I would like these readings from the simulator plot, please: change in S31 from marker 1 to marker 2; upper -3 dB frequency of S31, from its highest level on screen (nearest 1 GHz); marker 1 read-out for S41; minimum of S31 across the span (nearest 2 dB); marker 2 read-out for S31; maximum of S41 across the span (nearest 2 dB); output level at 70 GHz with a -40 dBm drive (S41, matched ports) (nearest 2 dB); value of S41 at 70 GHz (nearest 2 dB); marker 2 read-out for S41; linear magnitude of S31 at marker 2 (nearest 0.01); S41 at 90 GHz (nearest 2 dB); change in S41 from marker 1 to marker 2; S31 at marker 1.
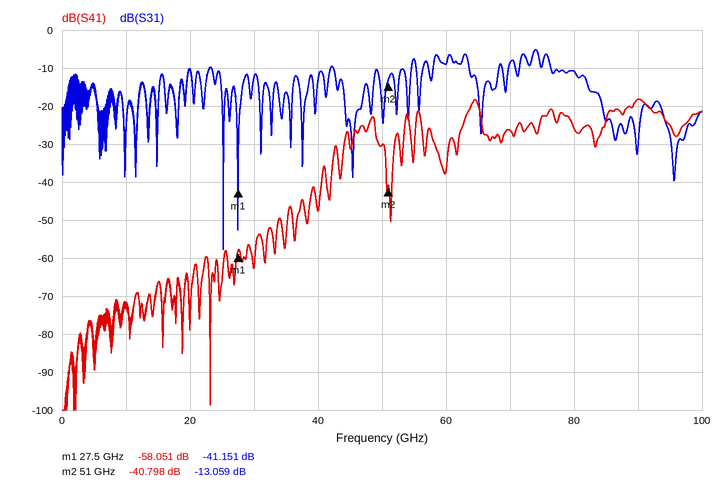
28.092 dB
75 GHz
-58.051 dB
-58 dB
-13.059 dB
-18 dB
-66 dBm
-26 dB
-40.798 dB
0.22
-18 dB
17.253 dB
-41.151 dB
